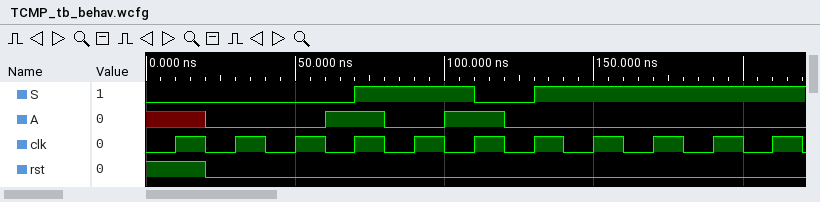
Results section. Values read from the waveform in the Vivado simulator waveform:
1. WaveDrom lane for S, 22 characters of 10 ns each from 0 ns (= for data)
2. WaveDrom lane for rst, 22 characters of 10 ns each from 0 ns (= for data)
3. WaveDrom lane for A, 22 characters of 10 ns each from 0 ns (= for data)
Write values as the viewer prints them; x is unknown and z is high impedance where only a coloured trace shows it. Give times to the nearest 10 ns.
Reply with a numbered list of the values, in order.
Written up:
1. {name: 'S', wave: '0......1...0.1........'}
2. {name: 'rst', wave: '1.0...................'}
3. {name: 'A', wave: 'x.0...1.0.1.0.........'}
